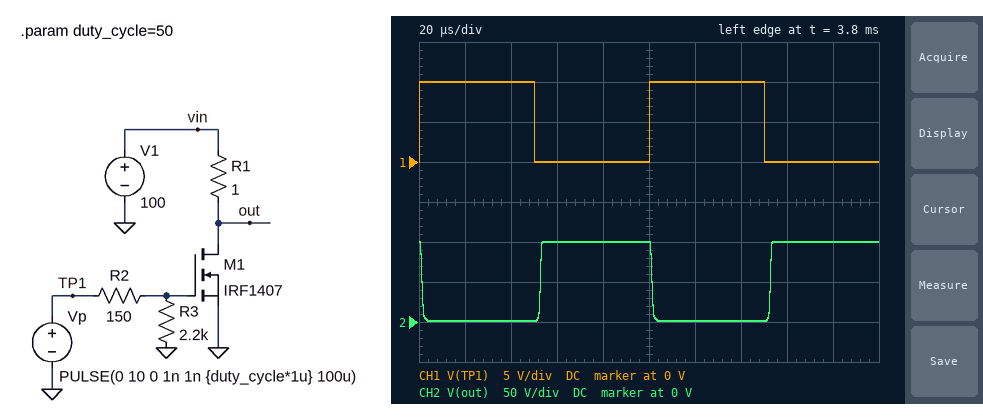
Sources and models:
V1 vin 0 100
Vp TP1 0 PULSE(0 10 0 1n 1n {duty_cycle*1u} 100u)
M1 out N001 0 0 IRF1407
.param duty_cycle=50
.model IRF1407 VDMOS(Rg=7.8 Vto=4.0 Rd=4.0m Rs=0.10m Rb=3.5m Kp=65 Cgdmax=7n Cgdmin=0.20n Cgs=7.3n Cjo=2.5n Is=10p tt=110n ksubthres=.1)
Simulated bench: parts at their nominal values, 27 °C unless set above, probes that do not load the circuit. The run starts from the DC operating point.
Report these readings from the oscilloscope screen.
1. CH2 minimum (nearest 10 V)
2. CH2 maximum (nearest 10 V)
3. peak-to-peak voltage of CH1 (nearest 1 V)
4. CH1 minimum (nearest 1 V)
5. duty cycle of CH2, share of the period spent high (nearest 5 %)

0 V
100 V
10 V
0 V
50 %
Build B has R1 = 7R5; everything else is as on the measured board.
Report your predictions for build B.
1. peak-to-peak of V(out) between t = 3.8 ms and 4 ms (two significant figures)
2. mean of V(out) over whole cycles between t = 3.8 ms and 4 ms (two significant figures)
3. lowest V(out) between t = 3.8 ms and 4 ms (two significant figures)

100 V
48 V
93 mV
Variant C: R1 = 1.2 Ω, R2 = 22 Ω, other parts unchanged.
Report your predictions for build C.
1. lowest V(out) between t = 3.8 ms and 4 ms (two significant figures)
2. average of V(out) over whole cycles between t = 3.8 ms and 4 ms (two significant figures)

560 mV
50 V
